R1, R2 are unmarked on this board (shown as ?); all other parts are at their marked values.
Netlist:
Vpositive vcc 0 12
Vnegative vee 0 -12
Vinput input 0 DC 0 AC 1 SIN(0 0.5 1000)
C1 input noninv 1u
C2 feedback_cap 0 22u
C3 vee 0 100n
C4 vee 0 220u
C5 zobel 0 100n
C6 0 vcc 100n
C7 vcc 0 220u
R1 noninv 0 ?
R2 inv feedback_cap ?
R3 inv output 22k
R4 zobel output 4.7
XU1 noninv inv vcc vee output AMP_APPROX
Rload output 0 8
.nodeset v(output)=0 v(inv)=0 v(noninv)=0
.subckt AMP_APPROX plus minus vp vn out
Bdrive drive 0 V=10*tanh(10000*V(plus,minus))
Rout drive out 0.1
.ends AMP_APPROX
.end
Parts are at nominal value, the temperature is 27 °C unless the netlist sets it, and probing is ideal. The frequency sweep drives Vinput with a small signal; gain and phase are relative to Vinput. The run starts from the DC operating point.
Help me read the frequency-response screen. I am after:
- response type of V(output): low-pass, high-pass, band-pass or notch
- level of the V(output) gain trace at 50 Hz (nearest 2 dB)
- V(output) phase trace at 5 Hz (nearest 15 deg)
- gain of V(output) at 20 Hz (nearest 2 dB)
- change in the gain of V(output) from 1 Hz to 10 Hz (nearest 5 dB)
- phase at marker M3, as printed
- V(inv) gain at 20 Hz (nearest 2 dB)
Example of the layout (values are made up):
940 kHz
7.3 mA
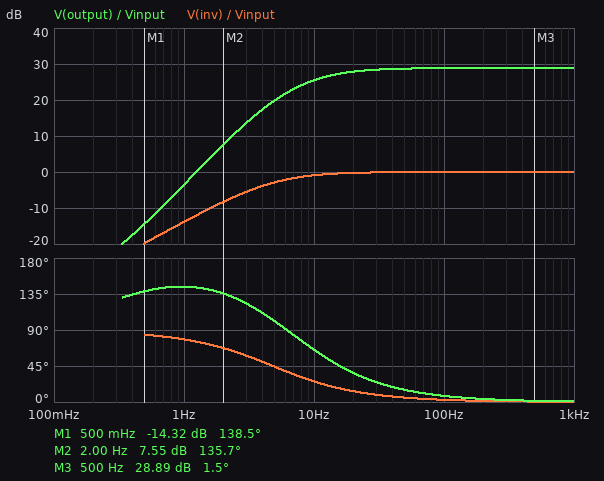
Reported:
high-pass
28 dB
105 deg
28 dB
30 dB
1.5 deg
0 dB
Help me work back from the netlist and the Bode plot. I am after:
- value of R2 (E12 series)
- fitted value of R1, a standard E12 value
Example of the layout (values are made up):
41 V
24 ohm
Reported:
820 Ω
33 kΩ
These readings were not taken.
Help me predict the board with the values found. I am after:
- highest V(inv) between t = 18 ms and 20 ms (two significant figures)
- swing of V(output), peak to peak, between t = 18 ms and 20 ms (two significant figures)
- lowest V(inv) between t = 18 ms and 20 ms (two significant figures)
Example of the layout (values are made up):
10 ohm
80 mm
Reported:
360 mV
20 V
-360 mV
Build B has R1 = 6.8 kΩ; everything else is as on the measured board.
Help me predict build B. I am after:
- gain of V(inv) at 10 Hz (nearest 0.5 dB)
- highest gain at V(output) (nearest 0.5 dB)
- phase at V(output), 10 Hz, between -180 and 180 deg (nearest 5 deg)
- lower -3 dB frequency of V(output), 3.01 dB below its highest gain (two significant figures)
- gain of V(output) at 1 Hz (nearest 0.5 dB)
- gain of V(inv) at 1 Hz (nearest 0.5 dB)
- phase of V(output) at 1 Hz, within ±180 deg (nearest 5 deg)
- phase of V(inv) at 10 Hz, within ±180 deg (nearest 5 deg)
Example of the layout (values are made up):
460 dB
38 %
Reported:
-8.0 dB
29.0 dB
105 deg
26 Hz
-17.0 dB
-27.5 dB
155 deg
65 deg
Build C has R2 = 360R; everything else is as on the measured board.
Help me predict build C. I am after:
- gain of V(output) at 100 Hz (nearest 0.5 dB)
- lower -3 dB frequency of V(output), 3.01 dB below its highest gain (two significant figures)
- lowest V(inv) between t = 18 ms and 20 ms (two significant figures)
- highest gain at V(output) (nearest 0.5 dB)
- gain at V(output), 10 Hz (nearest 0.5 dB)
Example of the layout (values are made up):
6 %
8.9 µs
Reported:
35.5 dB
21 Hz
-160 mV
36.0 dB
28.0 dB
